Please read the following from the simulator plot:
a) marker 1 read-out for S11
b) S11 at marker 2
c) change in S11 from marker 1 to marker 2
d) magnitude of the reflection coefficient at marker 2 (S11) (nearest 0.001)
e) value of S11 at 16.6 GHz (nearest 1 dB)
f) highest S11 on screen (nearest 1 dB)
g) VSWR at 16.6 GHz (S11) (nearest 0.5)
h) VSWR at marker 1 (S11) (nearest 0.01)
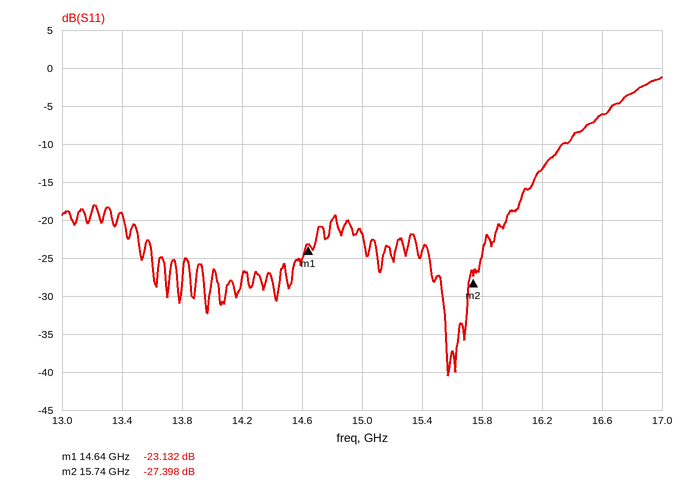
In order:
-23.132 dB
-27.398 dB
-4.266 dB
0.043
-6 dB
-1 dB
3.0
1.15
